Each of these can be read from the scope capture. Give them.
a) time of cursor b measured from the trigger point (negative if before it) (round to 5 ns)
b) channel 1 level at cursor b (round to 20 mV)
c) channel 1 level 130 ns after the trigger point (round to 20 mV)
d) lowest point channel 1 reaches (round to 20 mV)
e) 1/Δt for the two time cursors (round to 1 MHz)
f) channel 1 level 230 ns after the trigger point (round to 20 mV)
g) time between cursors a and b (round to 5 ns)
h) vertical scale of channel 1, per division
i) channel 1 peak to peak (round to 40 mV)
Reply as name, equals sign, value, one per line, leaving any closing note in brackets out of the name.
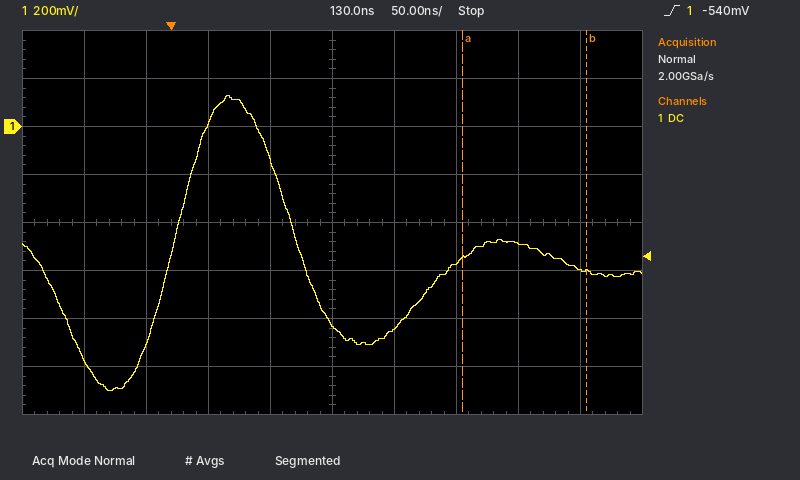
time of cursor b measured from the trigger point (negative if before it) = +335 ns
channel 1 level at cursor b = -600 mV
channel 1 level 130 ns after the trigger point = -820 mV
lowest point channel 1 reaches = -1.10 V
1/Δt for the two time cursors = 10 MHz
channel 1 level 230 ns after the trigger point = -560 mV
time between cursors a and b = 100 ns
vertical scale of channel 1, per division = 200 mV
channel 1 peak to peak = 1.24 V
